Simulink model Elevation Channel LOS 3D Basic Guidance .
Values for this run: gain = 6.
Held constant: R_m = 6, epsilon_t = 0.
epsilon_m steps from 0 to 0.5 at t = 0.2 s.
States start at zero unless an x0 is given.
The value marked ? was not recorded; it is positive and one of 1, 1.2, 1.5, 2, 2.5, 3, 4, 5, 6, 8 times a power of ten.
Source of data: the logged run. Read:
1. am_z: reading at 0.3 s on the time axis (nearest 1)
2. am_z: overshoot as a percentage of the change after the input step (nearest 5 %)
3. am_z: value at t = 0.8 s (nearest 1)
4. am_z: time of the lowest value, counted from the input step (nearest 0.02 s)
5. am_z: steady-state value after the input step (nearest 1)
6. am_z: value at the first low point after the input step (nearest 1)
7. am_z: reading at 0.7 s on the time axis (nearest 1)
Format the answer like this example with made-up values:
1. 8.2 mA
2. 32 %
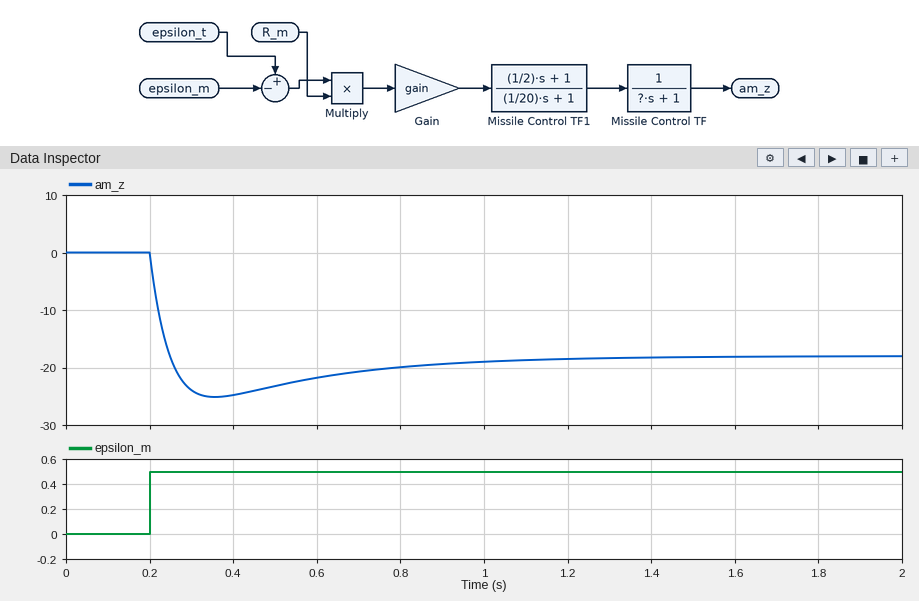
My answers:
1. -24
2. 40 %
3. -20
4. 0.16 s
5. -18
6. -25
7. -21
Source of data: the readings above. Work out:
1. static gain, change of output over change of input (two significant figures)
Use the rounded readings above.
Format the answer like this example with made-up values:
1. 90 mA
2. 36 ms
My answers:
1. -36
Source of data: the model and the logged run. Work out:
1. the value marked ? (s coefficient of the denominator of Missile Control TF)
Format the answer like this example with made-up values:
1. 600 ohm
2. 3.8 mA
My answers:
1. 0.3
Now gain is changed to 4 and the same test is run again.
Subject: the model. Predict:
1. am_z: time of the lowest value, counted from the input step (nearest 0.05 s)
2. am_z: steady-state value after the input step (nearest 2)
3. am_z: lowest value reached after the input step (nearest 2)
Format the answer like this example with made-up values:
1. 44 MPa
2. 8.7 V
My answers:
1. 0.15 s
2. -12
3. -16
